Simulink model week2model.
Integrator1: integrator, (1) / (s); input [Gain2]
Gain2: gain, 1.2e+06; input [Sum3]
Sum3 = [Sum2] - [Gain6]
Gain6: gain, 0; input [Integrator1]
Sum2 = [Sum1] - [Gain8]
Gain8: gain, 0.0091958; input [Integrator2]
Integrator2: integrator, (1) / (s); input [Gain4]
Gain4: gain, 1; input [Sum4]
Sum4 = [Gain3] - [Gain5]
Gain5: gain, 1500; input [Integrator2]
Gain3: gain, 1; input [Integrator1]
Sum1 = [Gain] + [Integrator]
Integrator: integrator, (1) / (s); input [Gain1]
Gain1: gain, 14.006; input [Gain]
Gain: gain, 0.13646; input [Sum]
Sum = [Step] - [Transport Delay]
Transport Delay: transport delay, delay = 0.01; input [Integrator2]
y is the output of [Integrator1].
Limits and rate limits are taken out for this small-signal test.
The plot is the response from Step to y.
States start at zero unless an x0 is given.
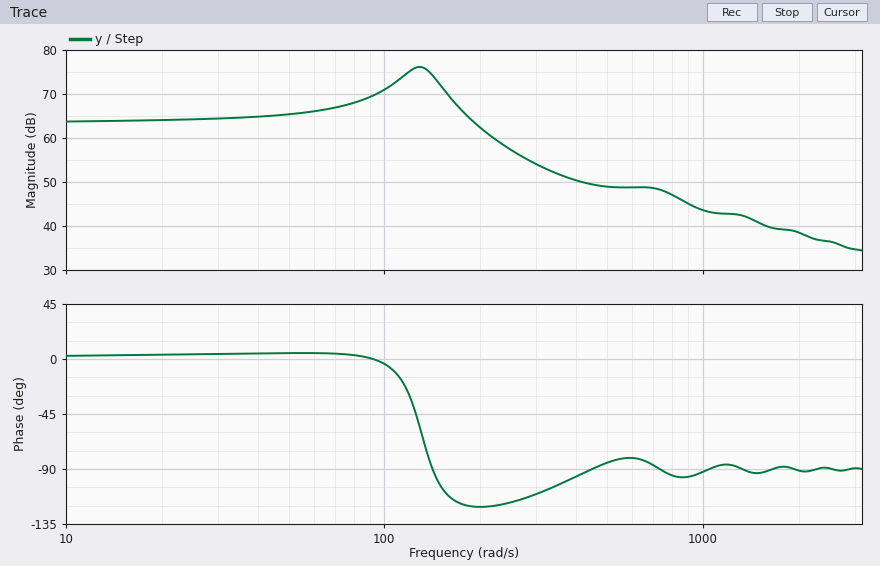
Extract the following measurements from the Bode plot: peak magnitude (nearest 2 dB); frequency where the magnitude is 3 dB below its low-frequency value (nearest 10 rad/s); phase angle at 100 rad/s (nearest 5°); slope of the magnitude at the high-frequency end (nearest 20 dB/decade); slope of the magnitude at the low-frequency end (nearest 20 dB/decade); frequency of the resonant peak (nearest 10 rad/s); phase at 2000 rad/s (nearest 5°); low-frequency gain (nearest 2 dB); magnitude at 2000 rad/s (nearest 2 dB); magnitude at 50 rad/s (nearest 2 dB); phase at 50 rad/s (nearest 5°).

76 dB
210 rad/s
-5°
-20 dB/decade
0 dB/decade
130 rad/s
-90°
64 dB
38 dB
66 dB
5°
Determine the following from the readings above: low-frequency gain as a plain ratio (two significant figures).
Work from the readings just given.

1600
